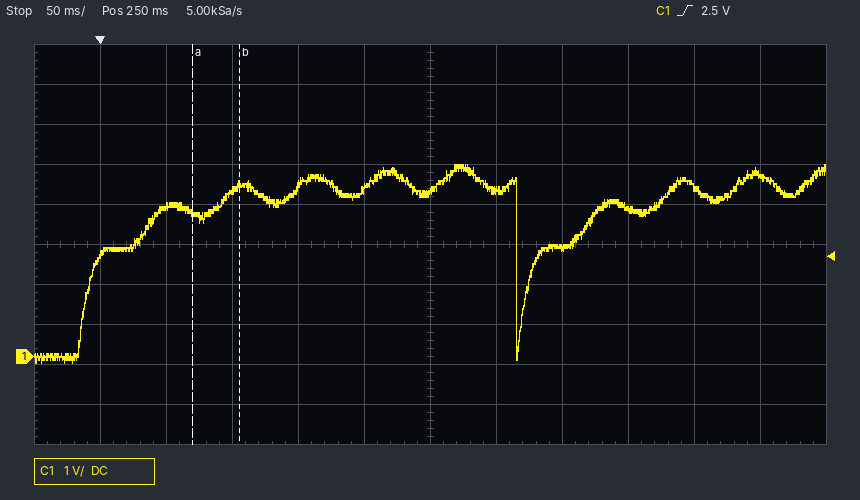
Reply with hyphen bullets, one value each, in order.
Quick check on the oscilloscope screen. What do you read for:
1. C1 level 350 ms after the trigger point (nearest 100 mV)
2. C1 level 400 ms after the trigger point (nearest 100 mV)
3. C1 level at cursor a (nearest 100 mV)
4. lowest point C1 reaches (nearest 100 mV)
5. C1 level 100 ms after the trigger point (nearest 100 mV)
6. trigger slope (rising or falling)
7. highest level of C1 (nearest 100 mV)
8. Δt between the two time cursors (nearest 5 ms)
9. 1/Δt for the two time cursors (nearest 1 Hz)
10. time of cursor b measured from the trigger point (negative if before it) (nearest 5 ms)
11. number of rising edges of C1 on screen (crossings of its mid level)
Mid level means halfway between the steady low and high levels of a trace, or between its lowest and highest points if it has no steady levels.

- 2.7 V
- 3.7 V
- 3.6 V
- -200 mV
- 4.2 V
- rising
- 4.8 V
- 35 ms
- 29 Hz
- +105 ms
- 2
